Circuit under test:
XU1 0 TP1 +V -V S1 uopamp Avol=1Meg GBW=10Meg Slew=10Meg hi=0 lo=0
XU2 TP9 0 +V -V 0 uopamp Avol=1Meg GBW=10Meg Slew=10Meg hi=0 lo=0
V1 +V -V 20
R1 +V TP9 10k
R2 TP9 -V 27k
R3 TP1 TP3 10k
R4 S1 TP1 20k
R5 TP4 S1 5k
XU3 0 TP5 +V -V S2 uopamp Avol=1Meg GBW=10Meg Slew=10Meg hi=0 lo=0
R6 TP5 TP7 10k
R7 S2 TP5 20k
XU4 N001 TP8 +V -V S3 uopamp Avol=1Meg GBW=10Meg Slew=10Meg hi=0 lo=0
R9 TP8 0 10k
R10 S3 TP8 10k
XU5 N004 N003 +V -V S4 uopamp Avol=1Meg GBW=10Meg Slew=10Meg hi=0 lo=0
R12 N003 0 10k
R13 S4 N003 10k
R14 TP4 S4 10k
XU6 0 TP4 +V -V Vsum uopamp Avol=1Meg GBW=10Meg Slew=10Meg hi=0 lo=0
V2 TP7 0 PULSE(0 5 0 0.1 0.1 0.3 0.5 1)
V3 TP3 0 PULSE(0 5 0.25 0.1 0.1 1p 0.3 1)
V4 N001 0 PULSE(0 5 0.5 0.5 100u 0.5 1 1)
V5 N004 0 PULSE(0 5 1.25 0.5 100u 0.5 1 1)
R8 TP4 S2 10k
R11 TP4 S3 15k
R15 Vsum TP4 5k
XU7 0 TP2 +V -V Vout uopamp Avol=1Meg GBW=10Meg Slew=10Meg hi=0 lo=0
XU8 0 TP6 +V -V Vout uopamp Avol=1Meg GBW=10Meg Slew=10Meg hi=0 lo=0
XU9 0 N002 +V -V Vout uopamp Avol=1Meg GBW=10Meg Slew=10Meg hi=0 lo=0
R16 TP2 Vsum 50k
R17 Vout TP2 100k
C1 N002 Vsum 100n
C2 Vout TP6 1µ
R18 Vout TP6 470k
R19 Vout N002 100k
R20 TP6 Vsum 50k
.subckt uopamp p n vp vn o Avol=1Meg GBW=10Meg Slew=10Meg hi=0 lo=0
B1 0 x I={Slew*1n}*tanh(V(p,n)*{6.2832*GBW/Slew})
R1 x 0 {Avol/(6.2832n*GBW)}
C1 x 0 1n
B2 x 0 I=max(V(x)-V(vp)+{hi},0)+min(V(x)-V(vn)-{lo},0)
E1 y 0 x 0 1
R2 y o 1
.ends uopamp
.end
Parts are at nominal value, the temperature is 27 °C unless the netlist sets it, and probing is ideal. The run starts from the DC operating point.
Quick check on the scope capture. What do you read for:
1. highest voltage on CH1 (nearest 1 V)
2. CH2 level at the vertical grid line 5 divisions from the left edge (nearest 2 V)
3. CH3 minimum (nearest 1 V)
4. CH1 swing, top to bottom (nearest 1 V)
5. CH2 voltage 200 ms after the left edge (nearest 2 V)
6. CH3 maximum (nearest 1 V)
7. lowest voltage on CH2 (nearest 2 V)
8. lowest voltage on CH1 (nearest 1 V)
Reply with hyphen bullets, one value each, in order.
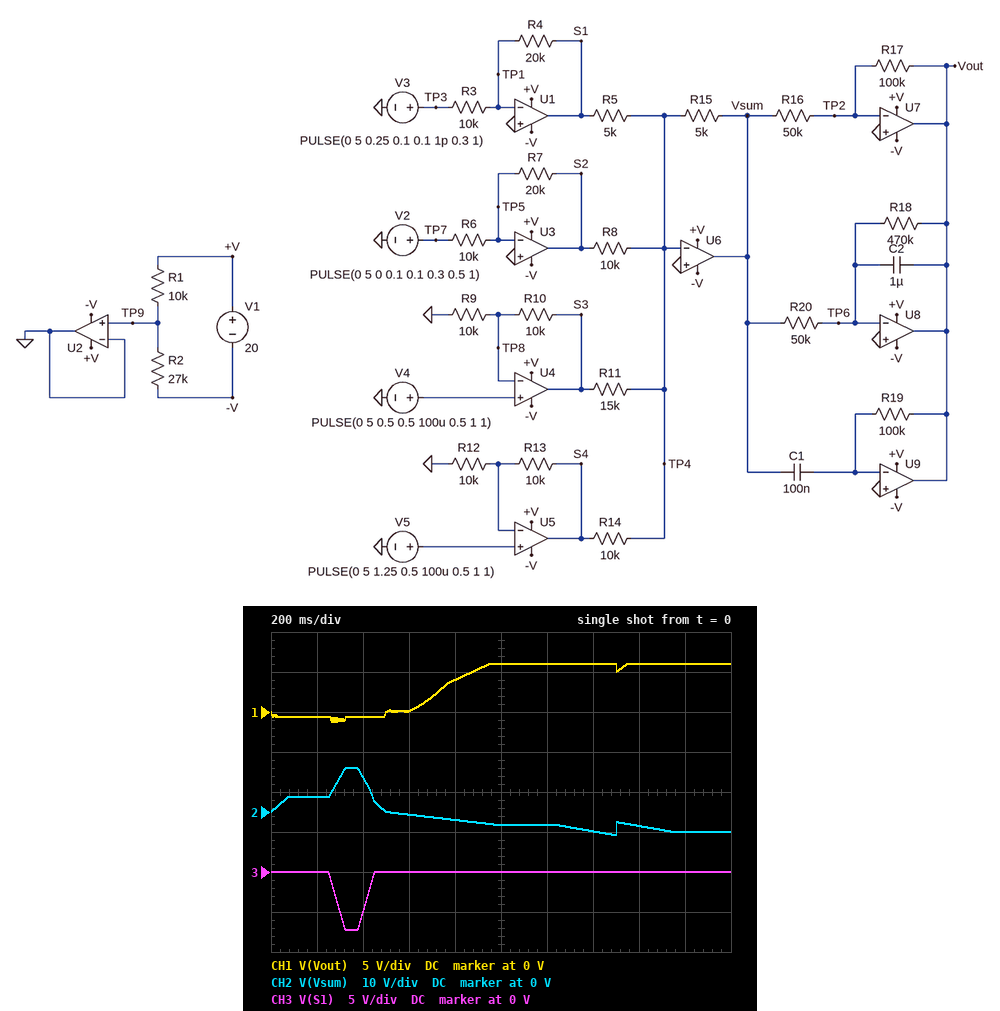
- 6 V
- -4 V
- -7 V
- 7 V
- 4 V
- 0 V
- -6 V
- -1 V
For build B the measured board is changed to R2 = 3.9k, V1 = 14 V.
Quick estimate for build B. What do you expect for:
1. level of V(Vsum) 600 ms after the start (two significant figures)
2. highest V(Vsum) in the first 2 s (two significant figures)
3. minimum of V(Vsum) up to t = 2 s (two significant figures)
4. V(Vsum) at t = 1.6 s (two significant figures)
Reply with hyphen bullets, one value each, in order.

- -3.3 mV
- 9.9 mV
- -8.3 mV
- -5.0 mV
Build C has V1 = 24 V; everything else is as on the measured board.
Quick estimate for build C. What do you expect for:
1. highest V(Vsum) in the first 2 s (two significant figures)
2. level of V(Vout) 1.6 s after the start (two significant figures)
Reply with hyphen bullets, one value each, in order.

- 13 V
- 7.0 V
